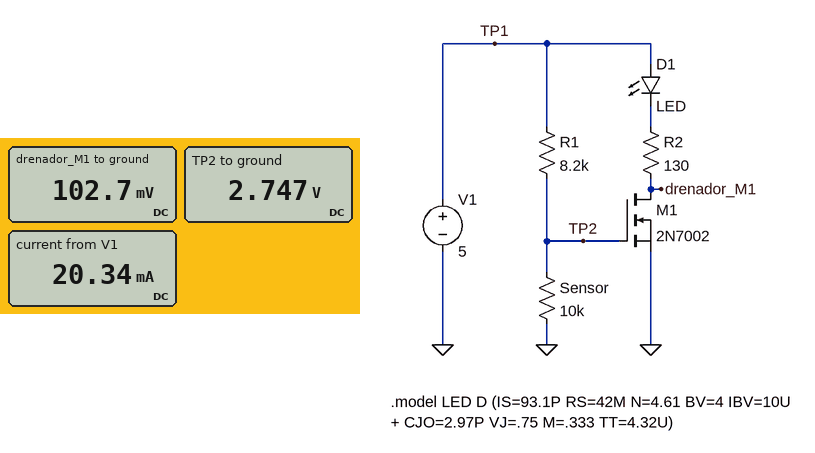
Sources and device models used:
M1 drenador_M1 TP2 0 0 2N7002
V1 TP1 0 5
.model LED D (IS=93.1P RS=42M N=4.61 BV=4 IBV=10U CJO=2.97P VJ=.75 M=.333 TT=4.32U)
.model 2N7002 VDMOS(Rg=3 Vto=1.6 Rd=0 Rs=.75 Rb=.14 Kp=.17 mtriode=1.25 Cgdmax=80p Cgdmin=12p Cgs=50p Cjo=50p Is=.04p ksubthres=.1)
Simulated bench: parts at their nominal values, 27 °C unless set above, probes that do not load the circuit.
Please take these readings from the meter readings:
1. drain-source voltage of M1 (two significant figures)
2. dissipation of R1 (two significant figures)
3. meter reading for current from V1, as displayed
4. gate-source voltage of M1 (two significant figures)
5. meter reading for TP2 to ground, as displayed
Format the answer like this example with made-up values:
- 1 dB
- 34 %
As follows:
- 100 mV
- 620 µW
- 20.34 mA
- 2.7 V
- 2.747 V
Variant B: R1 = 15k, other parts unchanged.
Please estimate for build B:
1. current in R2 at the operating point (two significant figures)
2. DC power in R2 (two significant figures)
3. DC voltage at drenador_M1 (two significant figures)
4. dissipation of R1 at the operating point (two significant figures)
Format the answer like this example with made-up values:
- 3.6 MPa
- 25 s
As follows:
- 13 mA
- 22 mW
- 1.1 V
- 600 µW
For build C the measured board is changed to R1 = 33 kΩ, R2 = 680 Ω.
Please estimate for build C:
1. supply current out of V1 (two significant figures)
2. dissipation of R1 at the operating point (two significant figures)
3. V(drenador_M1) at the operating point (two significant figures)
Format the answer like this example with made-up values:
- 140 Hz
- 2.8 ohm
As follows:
- 120 µA
- 450 µW
- 4.1 V
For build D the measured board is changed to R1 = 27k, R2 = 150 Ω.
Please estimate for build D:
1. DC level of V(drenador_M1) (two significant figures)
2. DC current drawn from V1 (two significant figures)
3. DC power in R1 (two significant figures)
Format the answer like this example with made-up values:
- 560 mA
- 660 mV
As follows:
- 3.7 V
- 140 µA
- 490 µW
